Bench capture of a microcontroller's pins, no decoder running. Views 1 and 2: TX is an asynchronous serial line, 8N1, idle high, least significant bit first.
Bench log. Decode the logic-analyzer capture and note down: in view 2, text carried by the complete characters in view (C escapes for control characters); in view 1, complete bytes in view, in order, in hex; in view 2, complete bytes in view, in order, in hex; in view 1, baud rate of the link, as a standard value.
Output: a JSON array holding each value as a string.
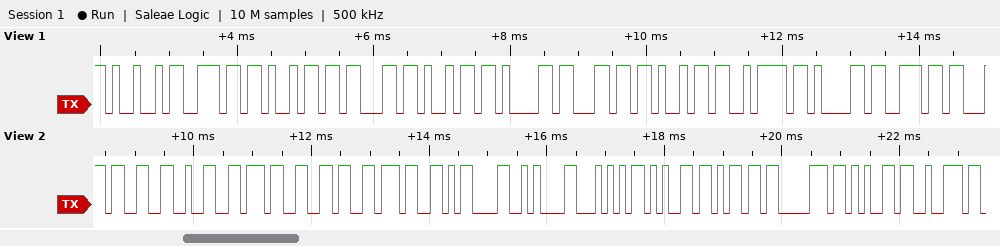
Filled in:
["\"32767\\r\\nTemper\"", "49 6E 69 63 69 61 6C 69 7A 61 6E", "33 32 37 36 37 0D 0A 54 65 6D 70 65 72", "9600 baud"]
